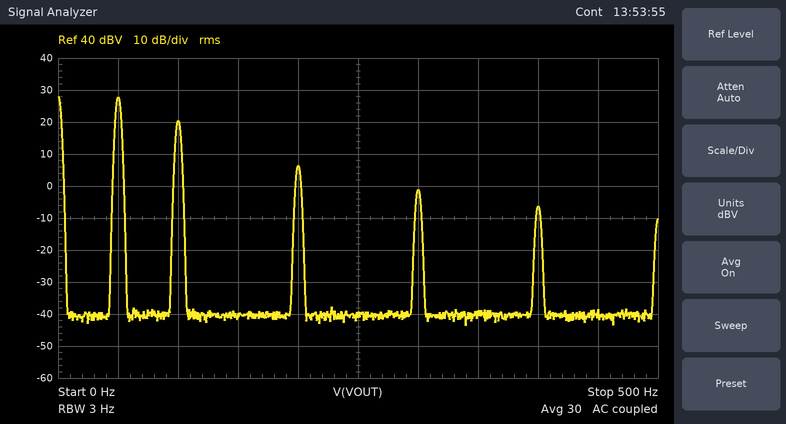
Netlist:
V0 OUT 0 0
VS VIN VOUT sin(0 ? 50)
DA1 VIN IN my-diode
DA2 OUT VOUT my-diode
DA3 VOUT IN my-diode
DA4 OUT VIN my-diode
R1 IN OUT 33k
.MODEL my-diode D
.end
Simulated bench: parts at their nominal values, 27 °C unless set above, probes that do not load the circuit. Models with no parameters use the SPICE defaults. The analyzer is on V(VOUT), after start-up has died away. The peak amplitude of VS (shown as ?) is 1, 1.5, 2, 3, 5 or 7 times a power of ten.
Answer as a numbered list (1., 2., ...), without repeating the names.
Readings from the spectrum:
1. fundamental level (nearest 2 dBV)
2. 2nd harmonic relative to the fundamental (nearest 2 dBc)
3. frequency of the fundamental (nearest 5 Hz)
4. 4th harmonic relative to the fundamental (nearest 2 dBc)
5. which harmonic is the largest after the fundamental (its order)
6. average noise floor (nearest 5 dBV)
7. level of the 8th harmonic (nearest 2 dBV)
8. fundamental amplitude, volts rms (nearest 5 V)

1. 28 dBV
2. -8 dBc
3. 50 Hz
4. -22 dBc
5. 2
6. -40 dBV
7. -6 dBV
8. 25 V
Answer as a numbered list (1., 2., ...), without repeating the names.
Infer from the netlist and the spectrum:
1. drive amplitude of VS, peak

1. 70 V
